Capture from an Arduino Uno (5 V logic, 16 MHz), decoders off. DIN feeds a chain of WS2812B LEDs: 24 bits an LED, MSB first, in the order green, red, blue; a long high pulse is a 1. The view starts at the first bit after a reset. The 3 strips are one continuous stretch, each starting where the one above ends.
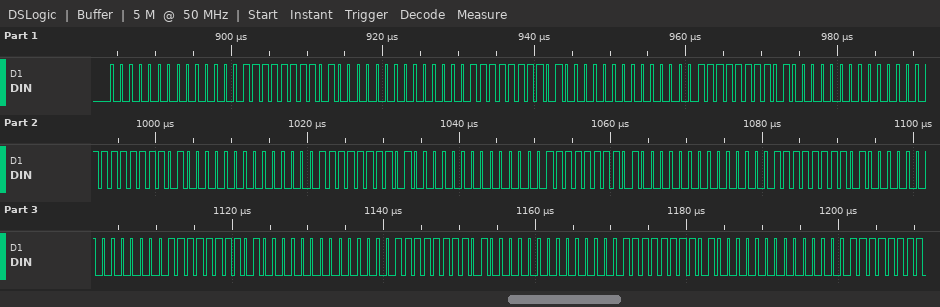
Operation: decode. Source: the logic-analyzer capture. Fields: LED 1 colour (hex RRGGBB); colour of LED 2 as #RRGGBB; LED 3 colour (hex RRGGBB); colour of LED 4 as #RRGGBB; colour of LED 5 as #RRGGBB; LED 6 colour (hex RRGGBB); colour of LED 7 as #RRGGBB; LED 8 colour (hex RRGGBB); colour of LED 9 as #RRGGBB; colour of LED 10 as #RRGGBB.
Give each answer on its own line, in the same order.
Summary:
#0300FD
#0300FD
#0300FD
#0300FD
#0300FD
#0300FD
#0300FD
#0300FD
#0300FD
#0300FD
